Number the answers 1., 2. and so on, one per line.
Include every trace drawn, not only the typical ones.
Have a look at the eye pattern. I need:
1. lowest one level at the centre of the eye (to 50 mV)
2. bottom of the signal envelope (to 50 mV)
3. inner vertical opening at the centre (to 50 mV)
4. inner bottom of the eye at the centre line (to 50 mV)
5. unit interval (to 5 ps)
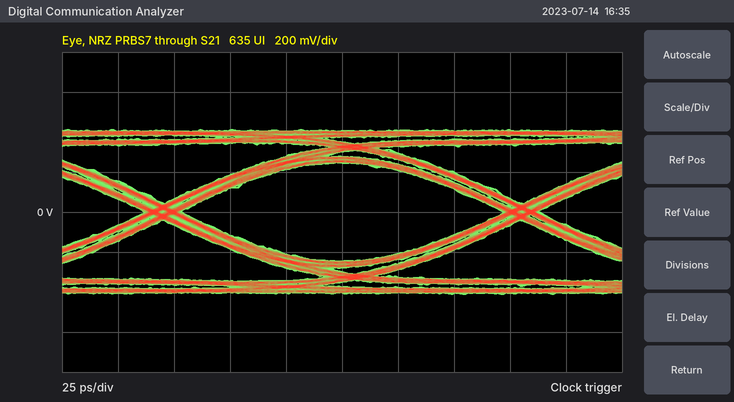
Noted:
1. 250 mV
2. -400 mV
3. 500 mV
4. -250 mV
5. 160 ps
